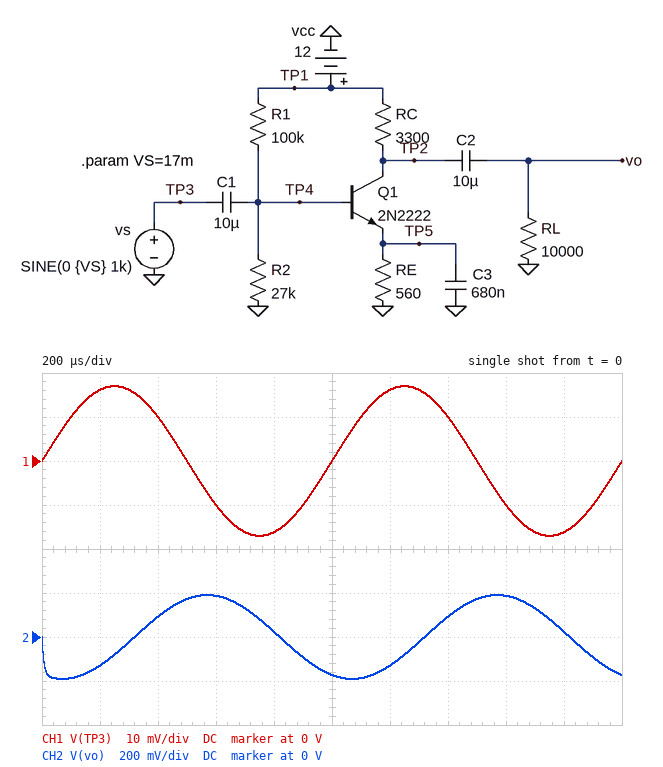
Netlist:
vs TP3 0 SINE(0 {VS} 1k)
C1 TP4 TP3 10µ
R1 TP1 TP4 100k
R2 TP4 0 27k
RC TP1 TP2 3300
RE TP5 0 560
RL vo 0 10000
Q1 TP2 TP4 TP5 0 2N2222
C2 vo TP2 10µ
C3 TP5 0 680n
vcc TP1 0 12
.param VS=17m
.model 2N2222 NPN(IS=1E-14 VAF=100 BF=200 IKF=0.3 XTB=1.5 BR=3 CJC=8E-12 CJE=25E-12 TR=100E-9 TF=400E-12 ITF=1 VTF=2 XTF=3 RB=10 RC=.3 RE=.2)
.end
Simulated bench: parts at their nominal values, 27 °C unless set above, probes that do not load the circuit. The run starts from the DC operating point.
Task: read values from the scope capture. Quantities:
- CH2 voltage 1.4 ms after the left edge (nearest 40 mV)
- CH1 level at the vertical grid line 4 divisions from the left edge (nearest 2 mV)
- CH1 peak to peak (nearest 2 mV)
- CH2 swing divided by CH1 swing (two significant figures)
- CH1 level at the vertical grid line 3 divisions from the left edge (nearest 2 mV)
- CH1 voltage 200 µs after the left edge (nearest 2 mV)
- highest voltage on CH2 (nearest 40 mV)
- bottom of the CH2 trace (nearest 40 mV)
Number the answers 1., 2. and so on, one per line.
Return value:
1. 80 mV
2. -16 mV
3. 34 mV
4. 11
5. -10 mV
6. 16 mV
7. 200 mV
8. -200 mV
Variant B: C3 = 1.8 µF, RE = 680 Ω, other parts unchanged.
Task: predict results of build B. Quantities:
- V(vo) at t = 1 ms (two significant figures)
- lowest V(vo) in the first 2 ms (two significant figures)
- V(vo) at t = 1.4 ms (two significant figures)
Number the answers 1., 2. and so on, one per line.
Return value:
1. -450 mV
2. -470 mV
3. 290 mV
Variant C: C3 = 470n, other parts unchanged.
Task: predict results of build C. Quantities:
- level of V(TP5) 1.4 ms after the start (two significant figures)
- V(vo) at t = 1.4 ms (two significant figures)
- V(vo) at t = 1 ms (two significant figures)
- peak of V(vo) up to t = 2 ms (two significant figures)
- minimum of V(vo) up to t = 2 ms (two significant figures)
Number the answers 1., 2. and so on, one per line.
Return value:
1. 1.6 V
2. 52 mV
3. -120 mV
4. 140 mV
5. -140 mV
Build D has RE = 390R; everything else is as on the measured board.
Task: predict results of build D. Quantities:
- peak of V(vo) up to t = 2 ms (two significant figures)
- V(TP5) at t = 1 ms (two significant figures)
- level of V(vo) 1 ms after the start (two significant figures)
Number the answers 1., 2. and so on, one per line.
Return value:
1. 180 mV
2. 1.3 V
3. -40 mV
